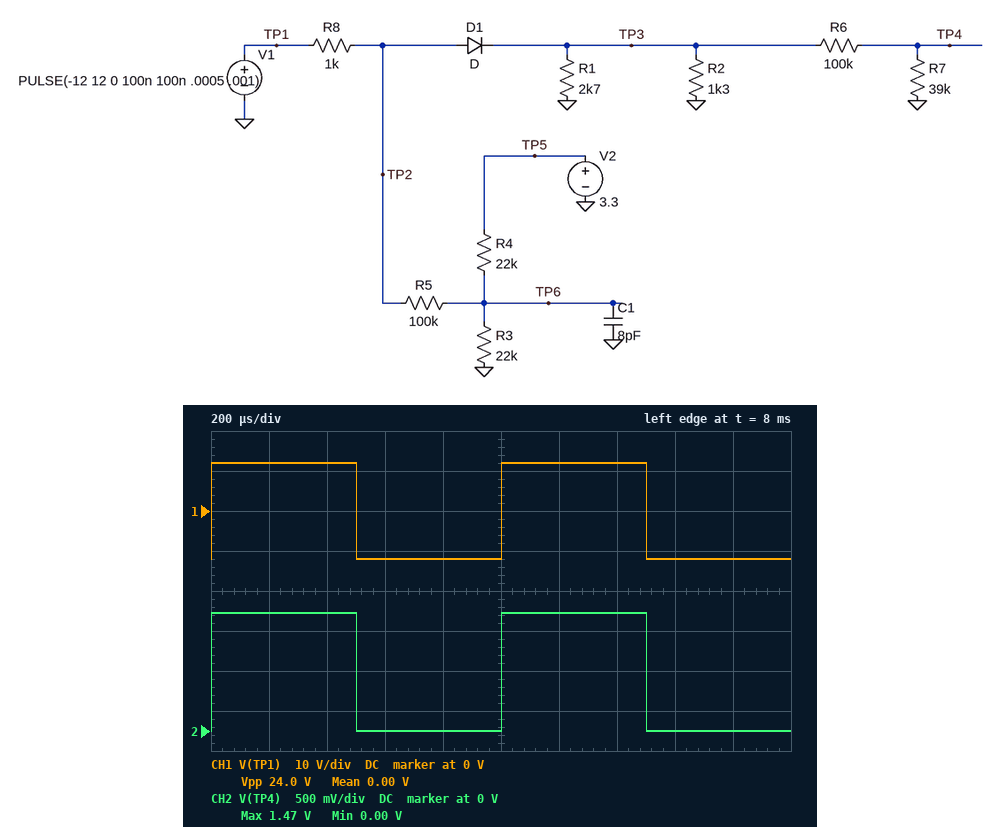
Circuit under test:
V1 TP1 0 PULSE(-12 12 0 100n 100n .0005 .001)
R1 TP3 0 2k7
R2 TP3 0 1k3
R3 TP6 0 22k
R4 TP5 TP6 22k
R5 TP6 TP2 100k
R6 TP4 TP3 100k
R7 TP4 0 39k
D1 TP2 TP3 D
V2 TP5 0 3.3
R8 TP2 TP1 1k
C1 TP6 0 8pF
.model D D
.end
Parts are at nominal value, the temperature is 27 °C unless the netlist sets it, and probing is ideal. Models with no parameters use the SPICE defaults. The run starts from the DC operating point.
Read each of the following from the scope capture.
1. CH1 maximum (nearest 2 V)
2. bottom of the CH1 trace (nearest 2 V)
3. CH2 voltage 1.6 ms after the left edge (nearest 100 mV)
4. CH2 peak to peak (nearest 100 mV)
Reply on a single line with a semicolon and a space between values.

12 V; -12 V; 0 V; 1.5 V
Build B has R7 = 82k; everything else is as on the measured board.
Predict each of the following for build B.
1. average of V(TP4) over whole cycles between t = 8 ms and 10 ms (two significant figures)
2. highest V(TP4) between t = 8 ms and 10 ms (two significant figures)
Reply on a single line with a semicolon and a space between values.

1.2 V; 2.4 V
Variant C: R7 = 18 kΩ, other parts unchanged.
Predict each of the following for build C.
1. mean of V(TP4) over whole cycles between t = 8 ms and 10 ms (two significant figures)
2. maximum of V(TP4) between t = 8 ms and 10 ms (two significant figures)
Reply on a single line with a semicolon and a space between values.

400 mV; 800 mV
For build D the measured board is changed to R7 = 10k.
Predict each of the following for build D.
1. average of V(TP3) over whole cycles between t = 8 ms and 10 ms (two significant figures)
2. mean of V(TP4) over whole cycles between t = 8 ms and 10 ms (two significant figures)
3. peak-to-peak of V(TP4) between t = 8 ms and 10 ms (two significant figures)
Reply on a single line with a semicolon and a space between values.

2.6 V; 240 mV; 480 mV
